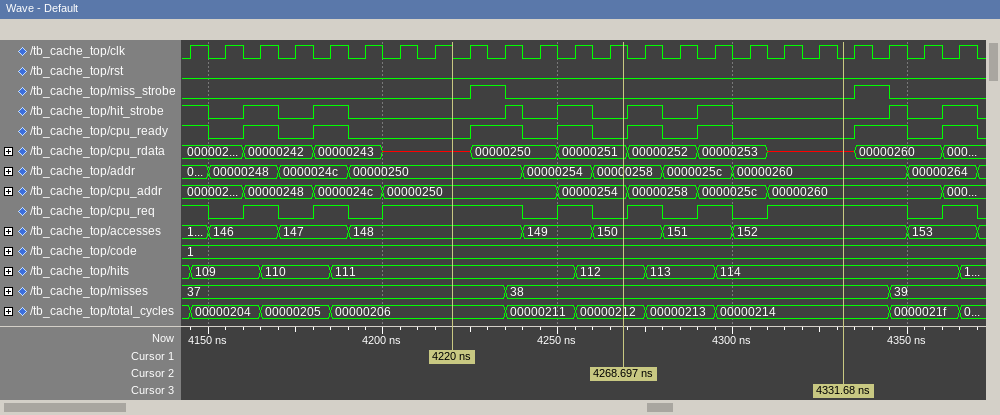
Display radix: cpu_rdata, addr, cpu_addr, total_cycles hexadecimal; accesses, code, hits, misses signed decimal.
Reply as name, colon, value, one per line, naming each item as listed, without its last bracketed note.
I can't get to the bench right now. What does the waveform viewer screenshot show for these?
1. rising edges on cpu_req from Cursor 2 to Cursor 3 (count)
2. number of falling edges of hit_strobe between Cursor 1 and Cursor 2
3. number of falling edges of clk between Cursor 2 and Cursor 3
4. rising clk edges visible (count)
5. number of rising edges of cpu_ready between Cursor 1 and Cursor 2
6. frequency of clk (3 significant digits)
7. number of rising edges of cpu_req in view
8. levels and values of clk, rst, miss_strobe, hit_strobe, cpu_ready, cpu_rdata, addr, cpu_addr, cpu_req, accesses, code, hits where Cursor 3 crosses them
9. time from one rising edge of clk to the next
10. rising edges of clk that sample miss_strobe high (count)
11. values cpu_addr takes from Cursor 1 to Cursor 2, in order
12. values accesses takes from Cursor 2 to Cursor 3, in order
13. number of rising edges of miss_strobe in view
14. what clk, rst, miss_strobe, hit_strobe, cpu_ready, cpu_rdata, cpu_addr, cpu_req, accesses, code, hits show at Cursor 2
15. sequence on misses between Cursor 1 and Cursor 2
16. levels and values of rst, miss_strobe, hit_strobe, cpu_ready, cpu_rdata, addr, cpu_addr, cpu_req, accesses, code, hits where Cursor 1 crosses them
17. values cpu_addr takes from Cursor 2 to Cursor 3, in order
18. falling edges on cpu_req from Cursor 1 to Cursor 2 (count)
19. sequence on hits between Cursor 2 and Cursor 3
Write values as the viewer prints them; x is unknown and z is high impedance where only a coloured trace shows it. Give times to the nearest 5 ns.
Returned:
rising edges on cpu_req from Cursor 2 to Cursor 3: 3
number of falling edges of hit_strobe between Cursor 1 and Cursor 2: 2
number of falling edges of clk between Cursor 2 and Cursor 3: 7
rising clk edges visible: 23
number of rising edges of cpu_ready between Cursor 1 and Cursor 2: 2
frequency of clk: 100 MHz
number of rising edges of cpu_req in view: 8
levels and values of clk, rst, miss_strobe, hit_strobe, cpu_ready, cpu_rdata, addr, cpu_addr, cpu_req, accesses, code, hits where Cursor 3 crosses them: clk=0, rst=0, miss_strobe=0, hit_strobe=0, cpu_ready=0, cpu_rdata=x, addr=00000260, cpu_addr=00000260, cpu_req=1, accesses=152, code=1, hits=114
time from one rising edge of clk to the next: 10 ns
rising edges of clk that sample miss_strobe high: 2
values cpu_addr takes from Cursor 1 to Cursor 2, in order: 00000250, 00000254
values accesses takes from Cursor 2 to Cursor 3, in order: 150, 151, 152
number of rising edges of miss_strobe in view: 2
what clk, rst, miss_strobe, hit_strobe, cpu_ready, cpu_rdata, cpu_addr, cpu_req, accesses, code, hits show at Cursor 2: clk=1, rst=0, miss_strobe=0, hit_strobe=0, cpu_ready=0, cpu_rdata=00000251, cpu_addr=00000254, cpu_req=0, accesses=150, code=1, hits=112
sequence on misses between Cursor 1 and Cursor 2: 37, 38
levels and values of rst, miss_strobe, hit_strobe, cpu_ready, cpu_rdata, addr, cpu_addr, cpu_req, accesses, code, hits where Cursor 1 crosses them: rst=0, miss_strobe=0, hit_strobe=0, cpu_ready=0, cpu_rdata=x, addr=00000250, cpu_addr=00000250, cpu_req=1, accesses=148, code=1, hits=111
values cpu_addr takes from Cursor 2 to Cursor 3, in order: 00000254, 00000258, 0000025c, 00000260
falling edges on cpu_req from Cursor 1 to Cursor 2: 2
sequence on hits between Cursor 2 and Cursor 3: 112, 113, 114
